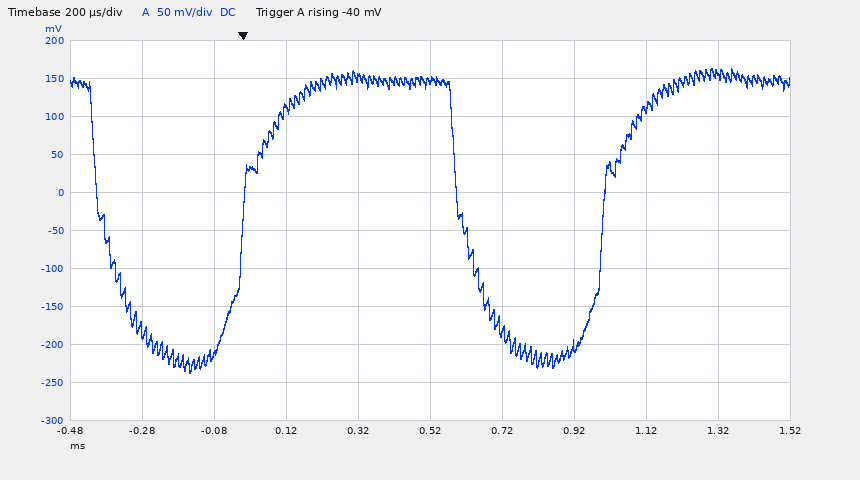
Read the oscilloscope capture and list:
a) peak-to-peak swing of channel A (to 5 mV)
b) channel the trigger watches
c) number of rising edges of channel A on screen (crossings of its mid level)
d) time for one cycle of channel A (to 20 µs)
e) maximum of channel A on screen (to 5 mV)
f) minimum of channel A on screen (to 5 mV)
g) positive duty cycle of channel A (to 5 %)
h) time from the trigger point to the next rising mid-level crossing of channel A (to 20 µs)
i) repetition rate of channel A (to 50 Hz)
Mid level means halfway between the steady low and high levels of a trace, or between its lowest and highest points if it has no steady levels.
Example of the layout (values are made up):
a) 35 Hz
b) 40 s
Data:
a) 400 mV
b) channel A
c) 2
d) 1.00 ms
e) 165 mV
f) -235 mV
g) 60 %
h) 1.00 ms
i) 1.00 kHz
